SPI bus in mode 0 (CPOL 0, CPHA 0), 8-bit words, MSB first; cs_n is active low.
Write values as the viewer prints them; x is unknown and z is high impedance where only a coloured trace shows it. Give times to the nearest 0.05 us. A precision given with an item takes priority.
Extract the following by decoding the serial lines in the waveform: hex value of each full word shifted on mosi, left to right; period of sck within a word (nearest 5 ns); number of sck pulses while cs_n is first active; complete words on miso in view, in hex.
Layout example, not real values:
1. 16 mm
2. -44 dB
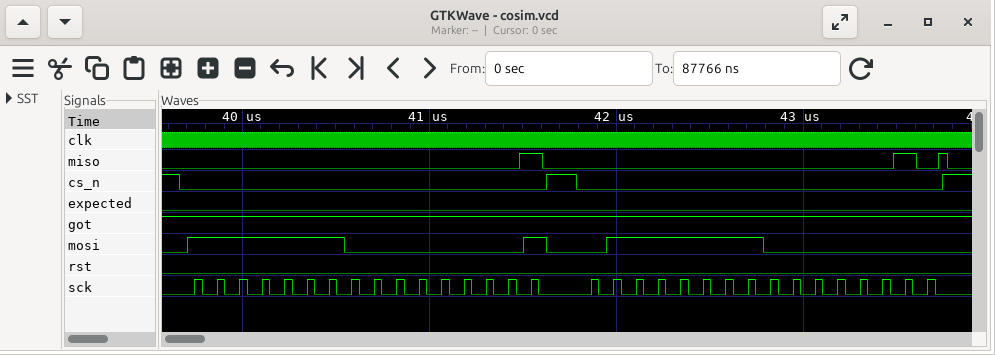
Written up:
1. FE, 01, 7F, 00
2. 120 ns
3. 16
4. 00, 01, 00, 02
